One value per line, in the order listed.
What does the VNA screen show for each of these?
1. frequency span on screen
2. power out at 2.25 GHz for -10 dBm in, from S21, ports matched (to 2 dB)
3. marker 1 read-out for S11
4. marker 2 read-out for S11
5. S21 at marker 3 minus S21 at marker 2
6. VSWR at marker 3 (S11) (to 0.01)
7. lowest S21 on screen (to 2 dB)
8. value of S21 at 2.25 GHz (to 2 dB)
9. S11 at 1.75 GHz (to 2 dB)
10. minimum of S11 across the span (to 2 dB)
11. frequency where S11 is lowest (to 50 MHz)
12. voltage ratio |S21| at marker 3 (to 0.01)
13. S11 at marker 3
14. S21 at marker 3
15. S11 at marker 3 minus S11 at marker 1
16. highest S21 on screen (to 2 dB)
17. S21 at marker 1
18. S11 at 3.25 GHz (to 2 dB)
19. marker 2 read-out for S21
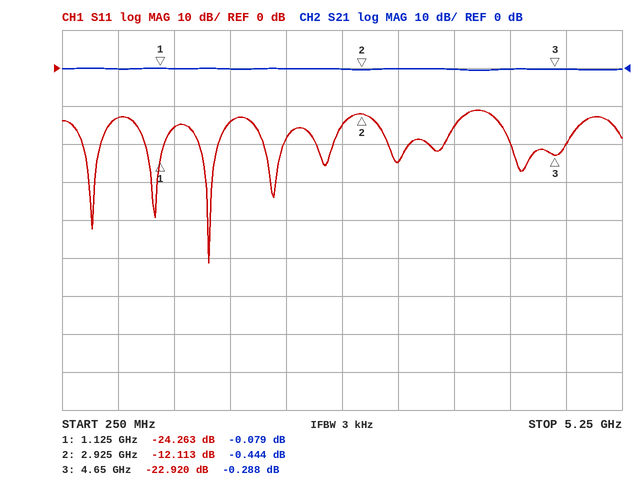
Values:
5 GHz
-10 dBm
-24.263 dB
-12.113 dB
0.156 dB
1.15
0 dB
0 dB
-14 dB
-52 dB
1.55 GHz
0.97
-22.920 dB
-0.288 dB
1.343 dB
0 dB
-0.079 dB
-24 dB
-0.444 dB
